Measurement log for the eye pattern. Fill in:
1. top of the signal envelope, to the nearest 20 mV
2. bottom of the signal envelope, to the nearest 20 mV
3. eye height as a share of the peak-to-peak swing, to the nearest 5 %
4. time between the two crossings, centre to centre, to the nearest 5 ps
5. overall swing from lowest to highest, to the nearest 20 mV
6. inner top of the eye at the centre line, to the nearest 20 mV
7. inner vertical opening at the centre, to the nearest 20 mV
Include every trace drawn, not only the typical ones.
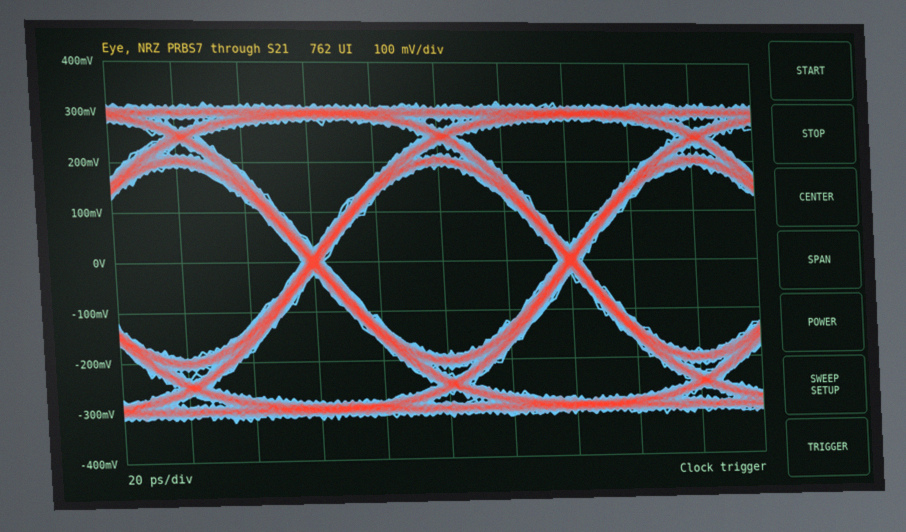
320 mV
-320 mV
60 %
80 ps
640 mV
200 mV
380 mV
